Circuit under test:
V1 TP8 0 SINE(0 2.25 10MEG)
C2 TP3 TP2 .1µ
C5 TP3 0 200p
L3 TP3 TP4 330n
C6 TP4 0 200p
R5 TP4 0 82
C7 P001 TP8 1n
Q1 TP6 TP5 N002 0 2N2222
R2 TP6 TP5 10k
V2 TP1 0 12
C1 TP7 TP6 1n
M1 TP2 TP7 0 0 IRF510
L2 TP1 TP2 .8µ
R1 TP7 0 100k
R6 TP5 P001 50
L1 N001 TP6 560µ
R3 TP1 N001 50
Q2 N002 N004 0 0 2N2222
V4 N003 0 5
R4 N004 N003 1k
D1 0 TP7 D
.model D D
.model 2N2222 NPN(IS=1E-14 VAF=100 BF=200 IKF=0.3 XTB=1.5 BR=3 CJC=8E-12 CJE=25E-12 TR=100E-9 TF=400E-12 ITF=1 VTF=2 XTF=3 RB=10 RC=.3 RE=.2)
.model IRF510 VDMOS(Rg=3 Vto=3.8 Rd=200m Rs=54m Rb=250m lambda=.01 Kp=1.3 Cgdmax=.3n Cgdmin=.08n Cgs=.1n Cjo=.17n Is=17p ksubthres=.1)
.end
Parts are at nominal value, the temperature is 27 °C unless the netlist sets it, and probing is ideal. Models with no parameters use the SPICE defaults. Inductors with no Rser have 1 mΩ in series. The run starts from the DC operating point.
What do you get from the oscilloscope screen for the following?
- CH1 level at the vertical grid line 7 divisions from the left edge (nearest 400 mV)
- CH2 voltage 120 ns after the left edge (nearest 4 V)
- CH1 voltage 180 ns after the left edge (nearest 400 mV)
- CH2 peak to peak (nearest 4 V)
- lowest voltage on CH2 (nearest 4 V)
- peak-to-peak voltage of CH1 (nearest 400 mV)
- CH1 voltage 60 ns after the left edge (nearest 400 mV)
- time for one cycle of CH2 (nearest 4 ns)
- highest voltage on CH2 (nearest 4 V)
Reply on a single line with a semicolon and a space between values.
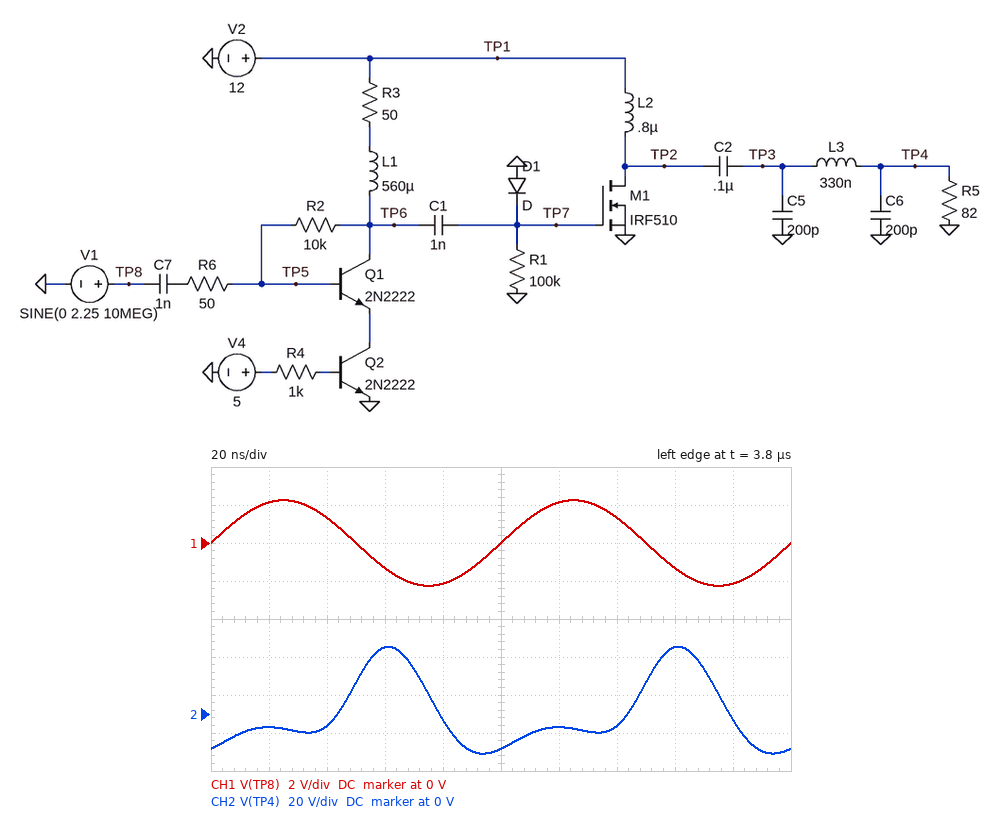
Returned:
1.2 V; -8 V; -2.0 V; 56 V; -20 V; 4.4 V; -1.2 V; 100 ns; 36 V
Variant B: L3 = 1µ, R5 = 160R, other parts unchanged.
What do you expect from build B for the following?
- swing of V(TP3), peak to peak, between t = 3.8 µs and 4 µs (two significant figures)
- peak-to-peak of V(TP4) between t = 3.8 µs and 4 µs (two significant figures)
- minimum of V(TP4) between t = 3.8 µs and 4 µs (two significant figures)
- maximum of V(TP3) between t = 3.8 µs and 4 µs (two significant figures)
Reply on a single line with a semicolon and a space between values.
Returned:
38 V; 74 V; -34 V; 27 V
